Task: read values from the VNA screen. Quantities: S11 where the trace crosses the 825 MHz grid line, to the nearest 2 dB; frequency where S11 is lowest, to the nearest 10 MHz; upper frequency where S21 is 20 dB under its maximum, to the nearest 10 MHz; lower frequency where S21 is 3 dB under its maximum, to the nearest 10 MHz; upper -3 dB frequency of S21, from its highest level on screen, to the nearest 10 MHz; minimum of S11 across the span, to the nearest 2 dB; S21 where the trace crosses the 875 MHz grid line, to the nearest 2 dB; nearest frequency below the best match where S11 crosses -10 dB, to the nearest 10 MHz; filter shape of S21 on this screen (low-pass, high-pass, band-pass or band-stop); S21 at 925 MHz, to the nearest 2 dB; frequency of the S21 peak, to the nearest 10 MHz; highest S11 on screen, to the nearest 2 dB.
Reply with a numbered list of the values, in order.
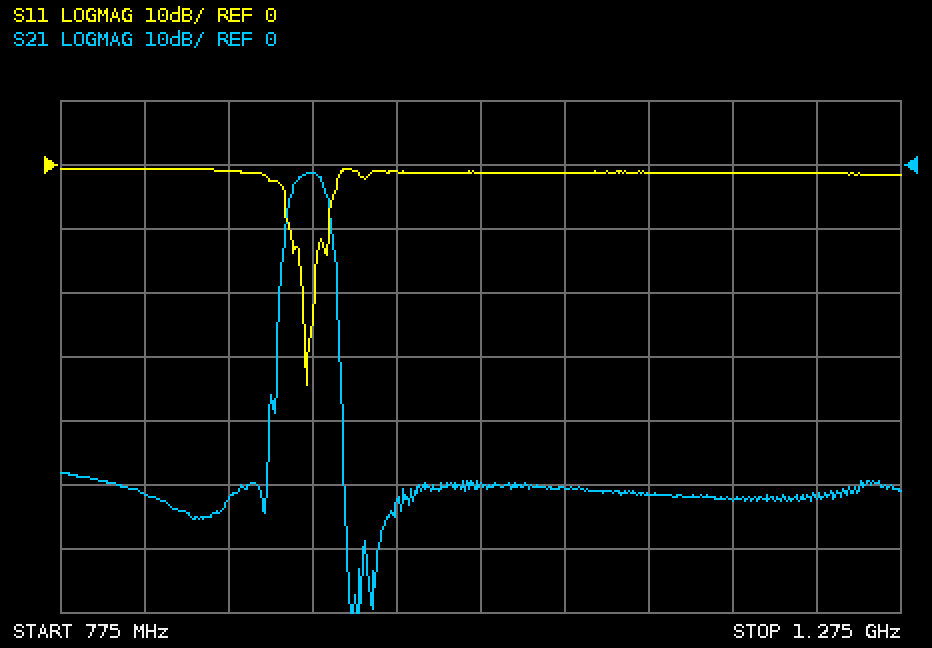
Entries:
1. 0 dB
2. 920 MHz
3. 940 MHz
4. 910 MHz
5. 930 MHz
6. -34 dB
7. -52 dB
8. 910 MHz
9. band-pass
10. -2 dB
11. 920 MHz
12. 0 dB
